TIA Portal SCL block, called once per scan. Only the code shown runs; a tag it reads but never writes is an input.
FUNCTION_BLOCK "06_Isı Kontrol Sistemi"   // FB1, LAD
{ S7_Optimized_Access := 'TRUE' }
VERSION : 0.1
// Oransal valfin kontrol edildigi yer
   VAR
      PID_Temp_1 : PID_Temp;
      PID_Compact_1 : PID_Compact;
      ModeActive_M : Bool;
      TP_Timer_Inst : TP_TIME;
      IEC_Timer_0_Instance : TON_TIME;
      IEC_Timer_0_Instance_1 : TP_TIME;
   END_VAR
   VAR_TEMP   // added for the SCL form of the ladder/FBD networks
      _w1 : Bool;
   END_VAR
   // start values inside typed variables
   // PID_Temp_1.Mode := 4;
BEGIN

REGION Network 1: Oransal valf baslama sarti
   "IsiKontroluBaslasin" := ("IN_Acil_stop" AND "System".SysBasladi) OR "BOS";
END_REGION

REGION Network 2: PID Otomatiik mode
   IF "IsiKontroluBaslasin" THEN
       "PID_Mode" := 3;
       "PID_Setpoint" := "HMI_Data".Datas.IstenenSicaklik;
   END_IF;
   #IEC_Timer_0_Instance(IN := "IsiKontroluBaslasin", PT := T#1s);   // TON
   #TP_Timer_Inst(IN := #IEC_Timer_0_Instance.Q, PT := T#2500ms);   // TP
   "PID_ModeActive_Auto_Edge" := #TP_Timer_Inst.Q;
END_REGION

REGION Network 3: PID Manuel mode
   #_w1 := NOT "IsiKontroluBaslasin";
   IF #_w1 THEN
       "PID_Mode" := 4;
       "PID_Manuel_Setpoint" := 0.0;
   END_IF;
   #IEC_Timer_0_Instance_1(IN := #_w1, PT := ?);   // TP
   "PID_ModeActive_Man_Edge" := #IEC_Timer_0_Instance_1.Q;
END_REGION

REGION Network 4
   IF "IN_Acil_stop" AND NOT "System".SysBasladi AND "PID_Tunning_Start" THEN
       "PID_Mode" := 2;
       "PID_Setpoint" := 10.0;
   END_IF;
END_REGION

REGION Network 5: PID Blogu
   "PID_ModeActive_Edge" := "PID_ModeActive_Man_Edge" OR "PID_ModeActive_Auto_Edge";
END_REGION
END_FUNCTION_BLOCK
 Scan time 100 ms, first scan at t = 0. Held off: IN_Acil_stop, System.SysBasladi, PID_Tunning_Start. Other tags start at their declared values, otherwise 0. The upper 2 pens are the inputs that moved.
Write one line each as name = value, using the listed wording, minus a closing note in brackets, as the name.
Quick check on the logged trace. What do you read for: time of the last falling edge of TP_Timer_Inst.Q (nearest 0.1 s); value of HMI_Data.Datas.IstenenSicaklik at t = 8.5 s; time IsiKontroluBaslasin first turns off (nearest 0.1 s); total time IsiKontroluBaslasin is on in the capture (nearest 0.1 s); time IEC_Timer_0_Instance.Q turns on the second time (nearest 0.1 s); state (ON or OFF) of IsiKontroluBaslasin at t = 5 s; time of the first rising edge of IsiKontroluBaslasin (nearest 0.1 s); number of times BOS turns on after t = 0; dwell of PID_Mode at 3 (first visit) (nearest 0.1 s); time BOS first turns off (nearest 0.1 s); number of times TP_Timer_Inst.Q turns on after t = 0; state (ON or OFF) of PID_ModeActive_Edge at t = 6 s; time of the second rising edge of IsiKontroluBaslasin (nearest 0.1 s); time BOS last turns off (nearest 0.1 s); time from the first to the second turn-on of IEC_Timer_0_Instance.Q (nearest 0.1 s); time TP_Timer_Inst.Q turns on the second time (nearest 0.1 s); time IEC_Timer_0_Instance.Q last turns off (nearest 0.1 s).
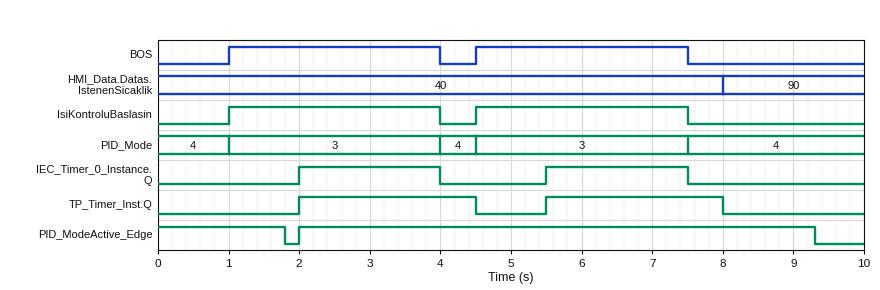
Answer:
time of the last falling edge of TP_Timer_Inst.Q = 8.0 s
value of HMI_Data.Datas.IstenenSicaklik at t = 8.5 s = 90
time IsiKontroluBaslasin first turns off = 4.0 s
total time IsiKontroluBaslasin is on in the capture = 6.0 s
time IEC_Timer_0_Instance.Q turns on the second time = 5.5 s
state (ON or OFF) of IsiKontroluBaslasin at t = 5 s = ON
time of the first rising edge of IsiKontroluBaslasin = 1.0 s
number of times BOS turns on after t = 0 = 2
dwell of PID_Mode at 3 (first visit) = 3.0 s
time BOS first turns off = 4.0 s
number of times TP_Timer_Inst.Q turns on after t = 0 = 2
state (ON or OFF) of PID_ModeActive_Edge at t = 6 s = ON
time of the second rising edge of IsiKontroluBaslasin = 4.5 s
time BOS last turns off = 7.5 s
time from the first to the second turn-on of IEC_Timer_0_Instance.Q = 3.5 s
time TP_Timer_Inst.Q turns on the second time = 5.5 s
time IEC_Timer_0_Instance.Q last turns off = 7.5 s
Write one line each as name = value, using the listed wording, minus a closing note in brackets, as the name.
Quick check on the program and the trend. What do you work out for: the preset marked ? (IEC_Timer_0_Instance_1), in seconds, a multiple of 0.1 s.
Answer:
the preset marked ? (IEC_Timer_0_Instance_1), in seconds, a multiple of 0.1 s = 1.8 s
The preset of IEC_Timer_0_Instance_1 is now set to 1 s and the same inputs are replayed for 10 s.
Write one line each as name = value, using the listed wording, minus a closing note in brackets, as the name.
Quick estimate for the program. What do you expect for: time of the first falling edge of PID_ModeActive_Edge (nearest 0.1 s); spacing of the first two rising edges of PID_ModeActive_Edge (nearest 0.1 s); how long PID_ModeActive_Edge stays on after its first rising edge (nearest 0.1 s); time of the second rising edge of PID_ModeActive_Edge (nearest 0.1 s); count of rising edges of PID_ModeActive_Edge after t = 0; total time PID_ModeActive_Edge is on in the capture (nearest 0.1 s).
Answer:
time of the first falling edge of PID_ModeActive_Edge = 1.0 s
spacing of the first two rising edges of PID_ModeActive_Edge = 3.5 s
how long PID_ModeActive_Edge stays on after its first rising edge = 3.0 s
time of the second rising edge of PID_ModeActive_Edge = 5.5 s
count of rising edges of PID_ModeActive_Edge after t = 0 = 2
total time PID_ModeActive_Edge is on in the capture = 7.0 s
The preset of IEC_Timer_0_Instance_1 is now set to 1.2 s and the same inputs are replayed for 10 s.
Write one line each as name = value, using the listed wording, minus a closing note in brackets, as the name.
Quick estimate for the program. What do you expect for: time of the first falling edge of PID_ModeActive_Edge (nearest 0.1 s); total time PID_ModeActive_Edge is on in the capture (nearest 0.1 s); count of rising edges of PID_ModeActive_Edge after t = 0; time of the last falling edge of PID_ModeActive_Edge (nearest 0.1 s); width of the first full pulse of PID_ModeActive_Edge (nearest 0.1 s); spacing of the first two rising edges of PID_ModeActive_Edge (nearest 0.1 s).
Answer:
time of the first falling edge of PID_ModeActive_Edge = 1.2 s
total time PID_ModeActive_Edge is on in the capture = 7.6 s
count of rising edges of PID_ModeActive_Edge after t = 0 = 2
time of the last falling edge of PID_ModeActive_Edge = 8.7 s
width of the first full pulse of PID_ModeActive_Edge = 3.2 s
spacing of the first two rising edges of PID_ModeActive_Edge = 3.5 s
